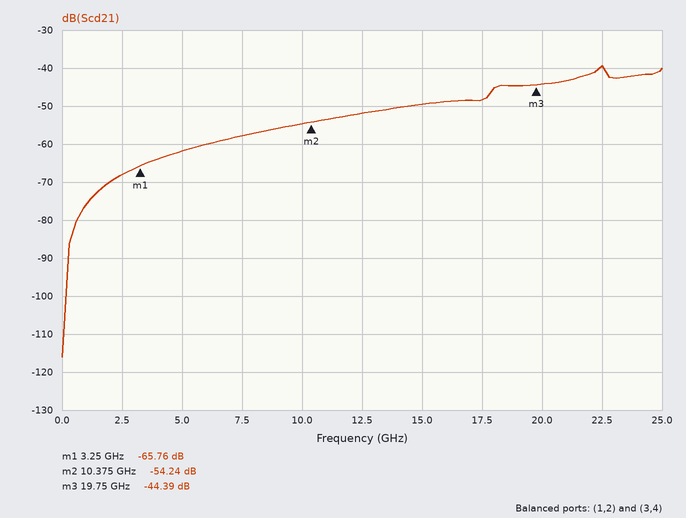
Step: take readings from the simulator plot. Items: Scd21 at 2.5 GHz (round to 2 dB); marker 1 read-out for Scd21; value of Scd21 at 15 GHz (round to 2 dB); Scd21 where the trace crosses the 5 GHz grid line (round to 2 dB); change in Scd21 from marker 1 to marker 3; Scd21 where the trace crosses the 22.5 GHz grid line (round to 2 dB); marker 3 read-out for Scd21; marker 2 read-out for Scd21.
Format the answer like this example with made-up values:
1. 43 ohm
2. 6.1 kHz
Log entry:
1. -68 dB
2. -65.76 dB
3. -50 dB
4. -62 dB
5. 21.37 dB
6. -40 dB
7. -44.39 dB
8. -54.24 dB
